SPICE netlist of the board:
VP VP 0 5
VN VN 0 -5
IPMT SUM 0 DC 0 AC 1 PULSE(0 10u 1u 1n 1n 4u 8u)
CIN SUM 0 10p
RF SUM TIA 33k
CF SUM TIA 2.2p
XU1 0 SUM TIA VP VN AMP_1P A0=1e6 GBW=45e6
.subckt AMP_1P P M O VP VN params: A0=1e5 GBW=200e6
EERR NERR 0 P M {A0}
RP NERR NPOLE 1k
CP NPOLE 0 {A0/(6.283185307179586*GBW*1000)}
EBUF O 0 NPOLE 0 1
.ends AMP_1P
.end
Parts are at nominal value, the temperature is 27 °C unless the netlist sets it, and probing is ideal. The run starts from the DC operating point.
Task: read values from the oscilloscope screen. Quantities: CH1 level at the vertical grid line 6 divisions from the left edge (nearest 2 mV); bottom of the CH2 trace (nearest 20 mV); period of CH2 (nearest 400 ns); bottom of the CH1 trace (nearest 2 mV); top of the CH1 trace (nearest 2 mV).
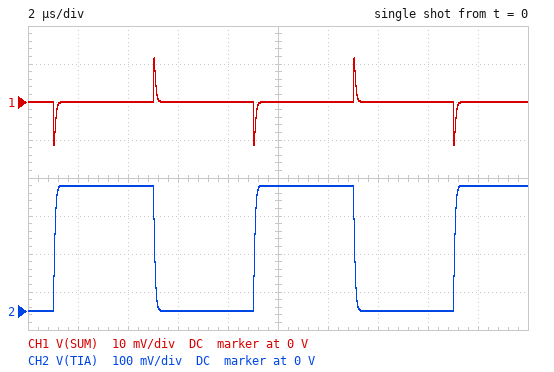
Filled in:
0 V
0 V
8.0 µs
-12 mV
12 mV
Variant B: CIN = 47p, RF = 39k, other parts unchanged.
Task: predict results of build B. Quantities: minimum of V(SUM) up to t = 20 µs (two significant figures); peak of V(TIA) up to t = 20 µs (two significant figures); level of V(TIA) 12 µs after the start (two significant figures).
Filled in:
-8.8 mV
440 mV
390 mV
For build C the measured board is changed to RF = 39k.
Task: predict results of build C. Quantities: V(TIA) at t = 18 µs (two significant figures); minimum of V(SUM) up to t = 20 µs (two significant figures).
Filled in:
390 mV
-12 mV
